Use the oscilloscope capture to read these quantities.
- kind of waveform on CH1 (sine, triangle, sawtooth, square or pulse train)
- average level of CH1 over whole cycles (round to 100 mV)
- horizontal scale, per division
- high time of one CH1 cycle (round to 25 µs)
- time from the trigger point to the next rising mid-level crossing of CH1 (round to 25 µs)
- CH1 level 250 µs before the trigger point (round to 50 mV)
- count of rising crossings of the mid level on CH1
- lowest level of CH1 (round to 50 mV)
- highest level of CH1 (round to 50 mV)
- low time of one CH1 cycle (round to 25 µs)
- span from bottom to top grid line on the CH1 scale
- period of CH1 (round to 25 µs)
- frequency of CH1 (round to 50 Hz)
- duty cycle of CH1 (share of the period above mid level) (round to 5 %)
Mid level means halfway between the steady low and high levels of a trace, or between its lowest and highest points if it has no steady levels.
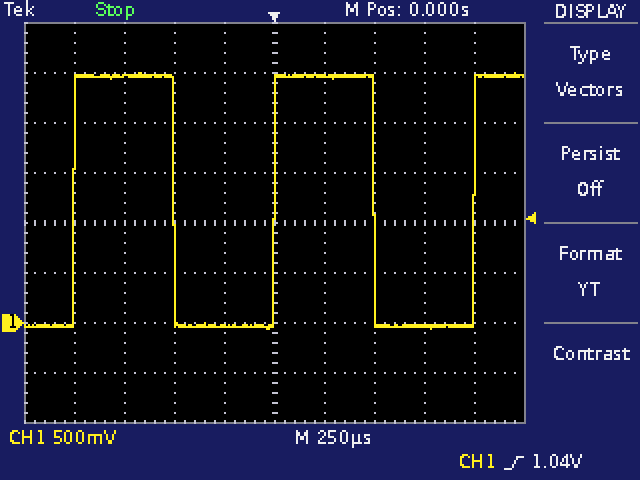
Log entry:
square
1.2 V
250 µs
500 µs
1.000 ms
-50 mV
3
-50 mV
2.50 V
500 µs
4 V
1.000 ms
1.00 kHz
50 %
